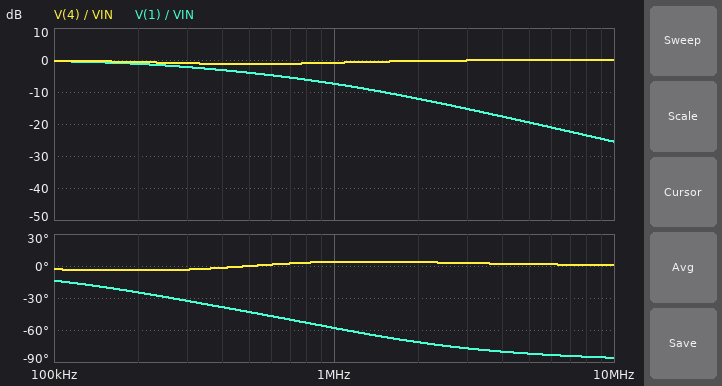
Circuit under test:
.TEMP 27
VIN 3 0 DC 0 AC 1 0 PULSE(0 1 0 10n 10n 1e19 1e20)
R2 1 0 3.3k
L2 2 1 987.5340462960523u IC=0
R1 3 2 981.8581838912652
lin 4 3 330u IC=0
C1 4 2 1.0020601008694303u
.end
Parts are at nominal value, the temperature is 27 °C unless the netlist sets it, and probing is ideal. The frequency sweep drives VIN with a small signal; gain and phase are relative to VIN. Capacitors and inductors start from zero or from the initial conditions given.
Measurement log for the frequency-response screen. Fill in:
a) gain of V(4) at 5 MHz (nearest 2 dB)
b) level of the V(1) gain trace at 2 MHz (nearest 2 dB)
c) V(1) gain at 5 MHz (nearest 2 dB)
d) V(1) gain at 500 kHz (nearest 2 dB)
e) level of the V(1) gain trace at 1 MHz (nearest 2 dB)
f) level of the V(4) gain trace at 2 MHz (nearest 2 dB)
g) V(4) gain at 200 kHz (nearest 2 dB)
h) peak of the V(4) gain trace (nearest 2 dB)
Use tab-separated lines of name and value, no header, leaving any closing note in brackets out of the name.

gain of V(4) at 5 MHz	0 dB
level of the V(1) gain trace at 2 MHz	-12 dB
V(1) gain at 5 MHz	-20 dB
V(1) gain at 500 kHz	-4 dB
level of the V(1) gain trace at 1 MHz	-8 dB
level of the V(4) gain trace at 2 MHz	0 dB
V(4) gain at 200 kHz	0 dB
peak of the V(4) gain trace	0 dB
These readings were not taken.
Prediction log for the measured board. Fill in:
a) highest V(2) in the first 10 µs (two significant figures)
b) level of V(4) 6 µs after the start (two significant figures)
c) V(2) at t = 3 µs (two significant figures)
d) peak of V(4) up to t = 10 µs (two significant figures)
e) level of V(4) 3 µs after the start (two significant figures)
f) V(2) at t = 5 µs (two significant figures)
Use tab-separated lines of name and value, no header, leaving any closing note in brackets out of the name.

highest V(2) in the first 10 µs	1.0 V
level of V(4) 6 µs after the start	1.0 V
V(2) at t = 3 µs	1.0 V
peak of V(4) up to t = 10 µs	1.0 V
level of V(4) 3 µs after the start	1.0 V
V(2) at t = 5 µs	1.0 V
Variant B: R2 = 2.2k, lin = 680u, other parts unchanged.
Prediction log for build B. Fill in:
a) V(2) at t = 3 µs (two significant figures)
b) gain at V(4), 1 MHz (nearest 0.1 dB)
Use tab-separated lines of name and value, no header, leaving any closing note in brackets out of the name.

V(2) at t = 3 µs	970 mV
gain at V(4), 1 MHz	-0.7 dB
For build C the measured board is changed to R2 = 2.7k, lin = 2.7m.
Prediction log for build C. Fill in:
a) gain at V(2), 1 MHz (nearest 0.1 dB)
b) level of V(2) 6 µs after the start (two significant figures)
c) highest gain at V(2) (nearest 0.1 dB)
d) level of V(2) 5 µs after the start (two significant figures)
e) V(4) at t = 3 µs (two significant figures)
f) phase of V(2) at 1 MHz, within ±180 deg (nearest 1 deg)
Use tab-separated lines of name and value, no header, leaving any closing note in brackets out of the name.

gain at V(2), 1 MHz	-0.6 dB
level of V(2) 6 µs after the start	940 mV
highest gain at V(2)	0 dB
level of V(2) 5 µs after the start	920 mV
V(4) at t = 3 µs	870 mV
phase of V(2) at 1 MHz, within ±180 deg	7 deg
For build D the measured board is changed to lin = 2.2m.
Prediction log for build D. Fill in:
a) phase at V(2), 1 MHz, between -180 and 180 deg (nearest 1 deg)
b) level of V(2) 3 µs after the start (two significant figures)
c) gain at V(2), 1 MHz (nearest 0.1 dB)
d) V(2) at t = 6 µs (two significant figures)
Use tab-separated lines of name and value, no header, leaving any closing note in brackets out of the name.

phase at V(2), 1 MHz, between -180 and 180 deg	6 deg
level of V(2) 3 µs after the start	910 mV
gain at V(2), 1 MHz	-0.7 dB
V(2) at t = 6 µs	970 mV
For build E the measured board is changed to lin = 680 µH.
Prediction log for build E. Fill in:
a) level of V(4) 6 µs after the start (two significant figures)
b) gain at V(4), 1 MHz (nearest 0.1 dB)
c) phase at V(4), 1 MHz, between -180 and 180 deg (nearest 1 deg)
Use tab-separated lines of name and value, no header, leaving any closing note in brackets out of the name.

level of V(4) 6 µs after the start	1.0 V
gain at V(4), 1 MHz	-0.8 dB
phase at V(4), 1 MHz, between -180 and 180 deg	5 deg
